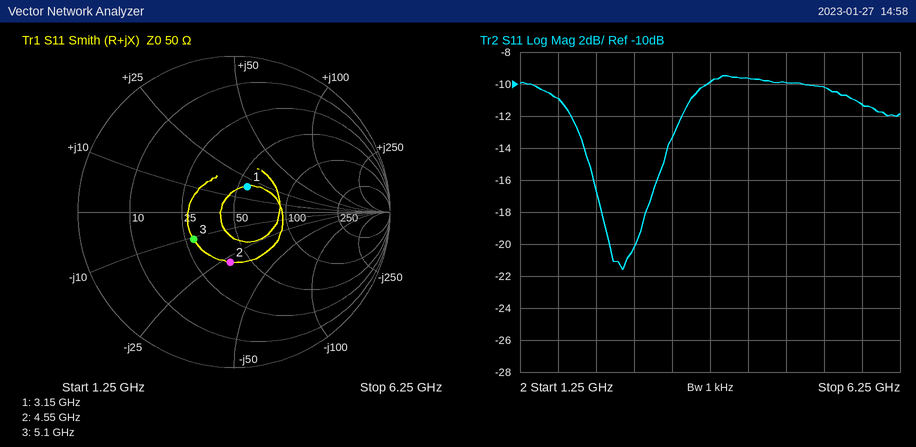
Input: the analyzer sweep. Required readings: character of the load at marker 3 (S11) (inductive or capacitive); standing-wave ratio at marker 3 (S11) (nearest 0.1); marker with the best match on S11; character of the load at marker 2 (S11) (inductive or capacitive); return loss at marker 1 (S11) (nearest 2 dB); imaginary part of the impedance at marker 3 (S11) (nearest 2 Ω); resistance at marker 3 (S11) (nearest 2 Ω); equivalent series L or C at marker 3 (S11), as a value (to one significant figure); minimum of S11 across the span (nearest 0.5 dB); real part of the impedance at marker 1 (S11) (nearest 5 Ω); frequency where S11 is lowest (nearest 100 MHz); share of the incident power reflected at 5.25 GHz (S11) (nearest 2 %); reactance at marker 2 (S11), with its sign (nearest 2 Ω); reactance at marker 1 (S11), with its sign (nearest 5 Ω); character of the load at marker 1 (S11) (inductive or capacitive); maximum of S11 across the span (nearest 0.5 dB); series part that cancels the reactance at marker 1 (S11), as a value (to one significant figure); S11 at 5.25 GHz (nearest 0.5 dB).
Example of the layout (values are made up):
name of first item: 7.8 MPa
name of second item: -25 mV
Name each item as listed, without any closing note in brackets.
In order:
character of the load at marker 3 (S11): capacitive
standing-wave ratio at marker 3 (S11): 1.9
marker with the best match on S11: marker 1
character of the load at marker 2 (S11): capacitive
return loss at marker 1 (S11): 14 dB
imaginary part of the impedance at marker 3 (S11): -10 Ω
resistance at marker 3 (S11): 28 Ω
equivalent series L or C at marker 3 (S11), as a value: 3 pF
minimum of S11 across the span: -21.5 dB
real part of the impedance at marker 1 (S11): 55 Ω
frequency where S11 is lowest: 2.6 GHz
share of the incident power reflected at 5.25 GHz (S11): 10 %
reactance at marker 2 (S11), with its sign: -28 Ω
reactance at marker 1 (S11), with its sign: +20 Ω
character of the load at marker 1 (S11): inductive
maximum of S11 across the span: -9.5 dB
series part that cancels the reactance at marker 1 (S11), as a value: 3 pF
S11 at 5.25 GHz: -10.0 dB
